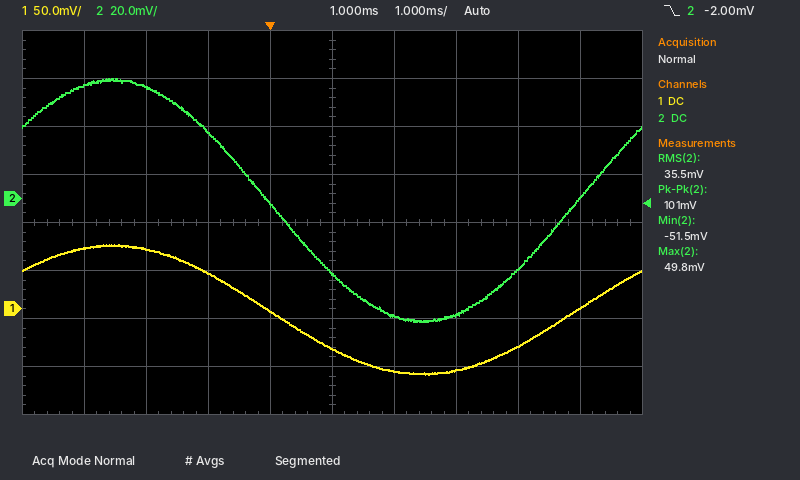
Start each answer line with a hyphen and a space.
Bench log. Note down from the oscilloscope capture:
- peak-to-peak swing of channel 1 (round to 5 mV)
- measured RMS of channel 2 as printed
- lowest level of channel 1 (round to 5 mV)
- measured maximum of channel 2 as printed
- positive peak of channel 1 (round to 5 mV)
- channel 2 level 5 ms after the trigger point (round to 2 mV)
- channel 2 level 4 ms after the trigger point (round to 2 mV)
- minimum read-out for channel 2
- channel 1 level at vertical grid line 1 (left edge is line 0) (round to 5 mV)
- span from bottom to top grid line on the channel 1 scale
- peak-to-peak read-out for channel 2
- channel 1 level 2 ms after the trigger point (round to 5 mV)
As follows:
- 135 mV
- 35.5 mV
- -70 mV
- 49.8 mV
- 65 mV
- 0 mV
- -30 mV
- -51.5 mV
- 65 mV
- 400 mV
- 101 mV
- -65 mV
